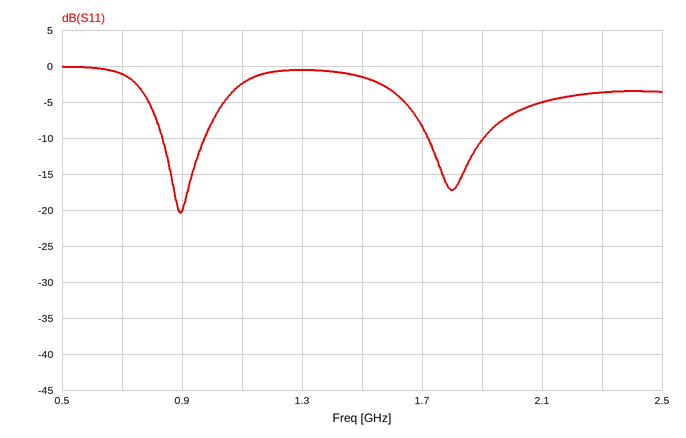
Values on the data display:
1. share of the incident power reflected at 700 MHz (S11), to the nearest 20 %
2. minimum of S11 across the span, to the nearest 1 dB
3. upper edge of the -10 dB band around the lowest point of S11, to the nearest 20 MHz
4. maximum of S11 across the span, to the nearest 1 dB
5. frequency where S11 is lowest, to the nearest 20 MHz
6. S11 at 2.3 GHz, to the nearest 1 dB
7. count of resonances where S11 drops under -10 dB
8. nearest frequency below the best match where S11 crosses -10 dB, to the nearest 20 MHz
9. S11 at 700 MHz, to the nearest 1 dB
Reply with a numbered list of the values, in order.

1. 80 %
2. -20 dB
3. 980 MHz
4. 0 dB
5. 900 MHz
6. -4 dB
7. 2
8. 840 MHz
9. -1 dB
